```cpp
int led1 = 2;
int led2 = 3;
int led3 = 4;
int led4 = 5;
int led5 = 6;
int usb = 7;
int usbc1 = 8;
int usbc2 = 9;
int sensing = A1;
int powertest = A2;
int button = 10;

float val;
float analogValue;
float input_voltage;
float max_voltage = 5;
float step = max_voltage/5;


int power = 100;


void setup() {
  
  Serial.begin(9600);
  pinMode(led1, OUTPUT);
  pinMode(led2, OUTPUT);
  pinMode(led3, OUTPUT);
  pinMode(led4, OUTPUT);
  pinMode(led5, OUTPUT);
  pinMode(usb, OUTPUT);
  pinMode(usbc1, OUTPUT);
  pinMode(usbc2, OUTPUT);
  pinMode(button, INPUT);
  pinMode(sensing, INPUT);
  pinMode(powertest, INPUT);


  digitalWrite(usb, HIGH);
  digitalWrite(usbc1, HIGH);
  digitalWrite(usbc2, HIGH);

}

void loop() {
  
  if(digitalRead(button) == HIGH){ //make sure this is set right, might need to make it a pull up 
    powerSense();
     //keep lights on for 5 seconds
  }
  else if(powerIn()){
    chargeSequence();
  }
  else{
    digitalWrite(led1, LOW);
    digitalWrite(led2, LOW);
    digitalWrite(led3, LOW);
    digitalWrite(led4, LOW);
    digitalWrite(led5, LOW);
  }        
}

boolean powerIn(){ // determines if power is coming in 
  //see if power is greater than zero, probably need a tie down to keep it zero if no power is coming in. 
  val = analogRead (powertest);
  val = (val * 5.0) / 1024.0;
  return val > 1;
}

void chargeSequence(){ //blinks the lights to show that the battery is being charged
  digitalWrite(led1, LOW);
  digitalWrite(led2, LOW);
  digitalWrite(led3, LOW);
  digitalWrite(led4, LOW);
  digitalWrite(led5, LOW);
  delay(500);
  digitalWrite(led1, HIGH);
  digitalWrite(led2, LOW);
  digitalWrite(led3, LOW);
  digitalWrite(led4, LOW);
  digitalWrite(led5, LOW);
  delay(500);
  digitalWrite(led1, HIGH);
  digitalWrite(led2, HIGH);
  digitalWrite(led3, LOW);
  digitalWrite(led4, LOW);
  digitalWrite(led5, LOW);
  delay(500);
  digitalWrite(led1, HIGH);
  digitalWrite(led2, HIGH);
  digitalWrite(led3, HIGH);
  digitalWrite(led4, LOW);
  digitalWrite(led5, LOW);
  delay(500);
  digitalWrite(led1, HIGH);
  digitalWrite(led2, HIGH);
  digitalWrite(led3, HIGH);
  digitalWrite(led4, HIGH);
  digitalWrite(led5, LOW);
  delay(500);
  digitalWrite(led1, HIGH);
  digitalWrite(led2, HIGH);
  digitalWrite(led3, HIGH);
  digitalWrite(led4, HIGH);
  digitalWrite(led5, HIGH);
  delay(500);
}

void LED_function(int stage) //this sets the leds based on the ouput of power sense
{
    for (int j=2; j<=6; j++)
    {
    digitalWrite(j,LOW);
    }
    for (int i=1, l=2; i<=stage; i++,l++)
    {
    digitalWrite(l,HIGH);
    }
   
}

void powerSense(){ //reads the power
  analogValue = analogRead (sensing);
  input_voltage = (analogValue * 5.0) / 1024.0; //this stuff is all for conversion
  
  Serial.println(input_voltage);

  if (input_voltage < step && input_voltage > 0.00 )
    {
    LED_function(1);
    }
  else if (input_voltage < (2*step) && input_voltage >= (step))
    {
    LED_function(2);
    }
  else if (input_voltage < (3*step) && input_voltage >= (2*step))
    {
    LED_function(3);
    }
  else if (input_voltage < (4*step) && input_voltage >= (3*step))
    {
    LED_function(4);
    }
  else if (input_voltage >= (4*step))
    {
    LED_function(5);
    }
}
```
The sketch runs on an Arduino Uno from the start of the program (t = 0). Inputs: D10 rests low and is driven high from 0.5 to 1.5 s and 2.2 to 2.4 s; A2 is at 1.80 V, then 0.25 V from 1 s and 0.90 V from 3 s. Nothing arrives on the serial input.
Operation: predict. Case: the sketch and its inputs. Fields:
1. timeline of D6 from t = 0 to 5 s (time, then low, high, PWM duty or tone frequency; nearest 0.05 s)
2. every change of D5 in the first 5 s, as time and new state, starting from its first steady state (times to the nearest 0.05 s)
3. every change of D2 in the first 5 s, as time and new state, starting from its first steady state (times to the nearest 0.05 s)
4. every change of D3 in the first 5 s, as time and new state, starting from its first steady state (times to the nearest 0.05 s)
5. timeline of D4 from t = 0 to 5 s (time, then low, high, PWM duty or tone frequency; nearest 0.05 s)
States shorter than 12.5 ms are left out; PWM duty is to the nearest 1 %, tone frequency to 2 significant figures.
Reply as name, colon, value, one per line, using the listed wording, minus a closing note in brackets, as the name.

timeline of D6 from t = 0 to 5 s: 0 s low; 2.5 s high; 3 s low
every change of D5 in the first 5 s, as time and new state, starting from its first steady state: 0 s low; 2 s high; 3 s low
every change of D2 in the first 5 s, as time and new state, starting from its first steady state: 0 s low; 0.5 s high; 3 s low
every change of D3 in the first 5 s, as time and new state, starting from its first steady state: 0 s low; 1 s high; 3 s low
timeline of D4 from t = 0 to 5 s: 0 s low; 1.5 s high; 3 s low
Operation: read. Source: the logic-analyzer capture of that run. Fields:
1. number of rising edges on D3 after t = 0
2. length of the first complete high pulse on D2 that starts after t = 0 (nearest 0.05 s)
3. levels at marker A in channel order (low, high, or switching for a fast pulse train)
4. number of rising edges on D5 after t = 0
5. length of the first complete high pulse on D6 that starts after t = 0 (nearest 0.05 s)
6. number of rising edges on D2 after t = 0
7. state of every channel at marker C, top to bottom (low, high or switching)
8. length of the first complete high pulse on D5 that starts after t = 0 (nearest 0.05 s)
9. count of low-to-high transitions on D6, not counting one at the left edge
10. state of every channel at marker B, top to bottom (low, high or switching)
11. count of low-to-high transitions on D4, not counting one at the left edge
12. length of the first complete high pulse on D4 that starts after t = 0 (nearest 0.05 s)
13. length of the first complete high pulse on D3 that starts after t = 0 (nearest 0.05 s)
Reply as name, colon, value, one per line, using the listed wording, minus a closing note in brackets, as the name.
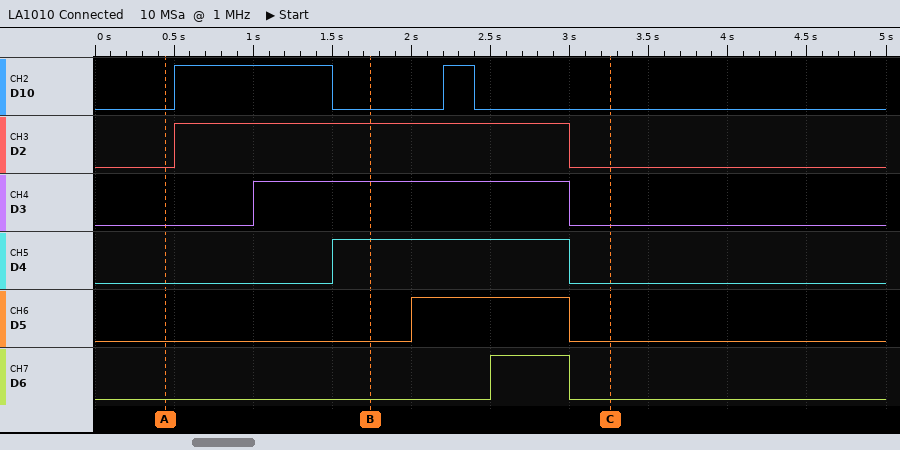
number of rising edges on D3 after t = 0: 1
length of the first complete high pulse on D2 that starts after t = 0: 2.50 s
levels at marker A in channel order: D10 low, D2 low, D3 low, D4 low, D5 low, D6 low
number of rising edges on D5 after t = 0: 1
length of the first complete high pulse on D6 that starts after t = 0: 0.50 s
number of rising edges on D2 after t = 0: 1
state of every channel at marker C, top to bottom: D10 low, D2 low, D3 low, D4 low, D5 low, D6 low
length of the first complete high pulse on D5 that starts after t = 0: 1.00 s
count of low-to-high transitions on D6, not counting one at the left edge: 1
state of every channel at marker B, top to bottom: D10 low, D2 high, D3 high, D4 high, D5 low, D6 low
count of low-to-high transitions on D4, not counting one at the left edge: 1
length of the first complete high pulse on D4 that starts after t = 0: 1.50 s
length of the first complete high pulse on D3 that starts after t = 0: 2.00 s
